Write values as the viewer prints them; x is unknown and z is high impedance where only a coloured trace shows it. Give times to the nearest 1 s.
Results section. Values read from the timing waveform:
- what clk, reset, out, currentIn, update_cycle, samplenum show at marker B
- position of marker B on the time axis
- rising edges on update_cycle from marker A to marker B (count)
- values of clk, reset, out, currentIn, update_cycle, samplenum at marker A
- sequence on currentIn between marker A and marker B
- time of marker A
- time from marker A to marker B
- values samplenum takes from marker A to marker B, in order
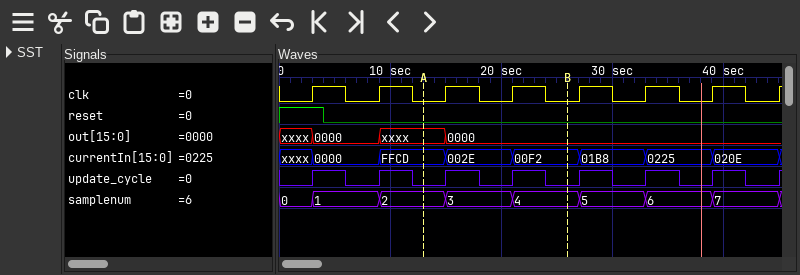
clk=0, reset=0, out=0000, currentIn=00F2, update_cycle=0, samplenum=4
26 s
2
clk=0, reset=0, out=xxxx, currentIn=FFCD, update_cycle=0, samplenum=2
FFCD, 002E, 00F2
13 s
13 s
2, 3, 4
